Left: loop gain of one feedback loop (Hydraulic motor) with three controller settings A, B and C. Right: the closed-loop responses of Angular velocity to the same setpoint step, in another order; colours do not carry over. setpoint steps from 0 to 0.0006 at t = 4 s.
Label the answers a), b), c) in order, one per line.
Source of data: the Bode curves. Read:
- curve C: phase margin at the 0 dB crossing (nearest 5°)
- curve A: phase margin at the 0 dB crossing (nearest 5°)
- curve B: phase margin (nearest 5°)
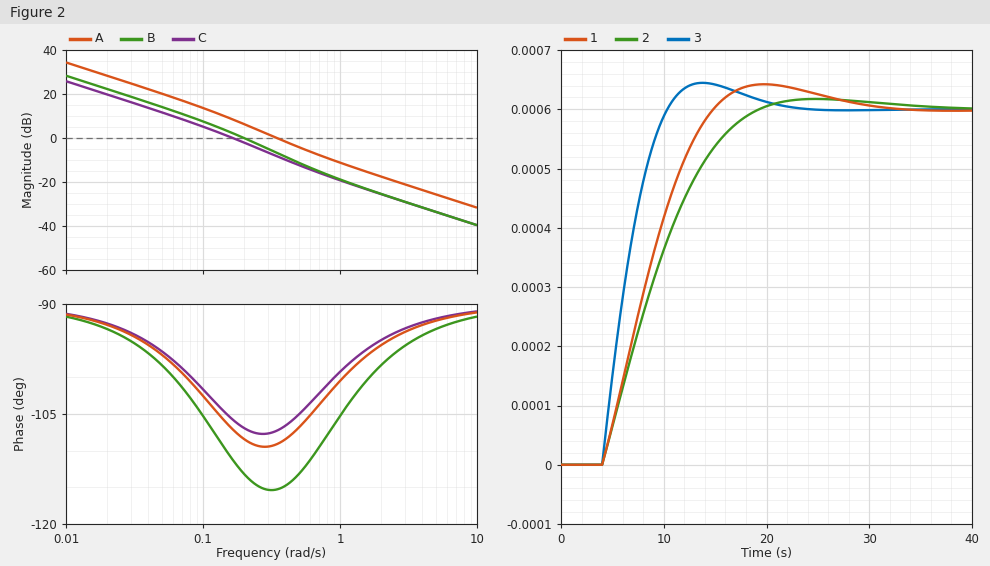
a) 75°
b) 70°
c) 65°
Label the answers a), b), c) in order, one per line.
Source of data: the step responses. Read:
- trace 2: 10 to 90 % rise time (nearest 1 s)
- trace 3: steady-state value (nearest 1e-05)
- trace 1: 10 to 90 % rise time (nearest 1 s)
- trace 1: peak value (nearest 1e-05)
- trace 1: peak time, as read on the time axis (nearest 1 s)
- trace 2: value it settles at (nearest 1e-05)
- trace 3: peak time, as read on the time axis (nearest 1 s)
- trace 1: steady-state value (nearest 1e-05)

a) 10 s
b) 0.00060
c) 8 s
d) 0.00064
e) 20 s
f) 0.00060
g) 14 s
h) 0.00060
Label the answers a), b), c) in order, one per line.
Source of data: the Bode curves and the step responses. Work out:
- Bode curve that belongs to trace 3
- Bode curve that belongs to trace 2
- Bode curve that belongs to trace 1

a) A
b) C
c) B
